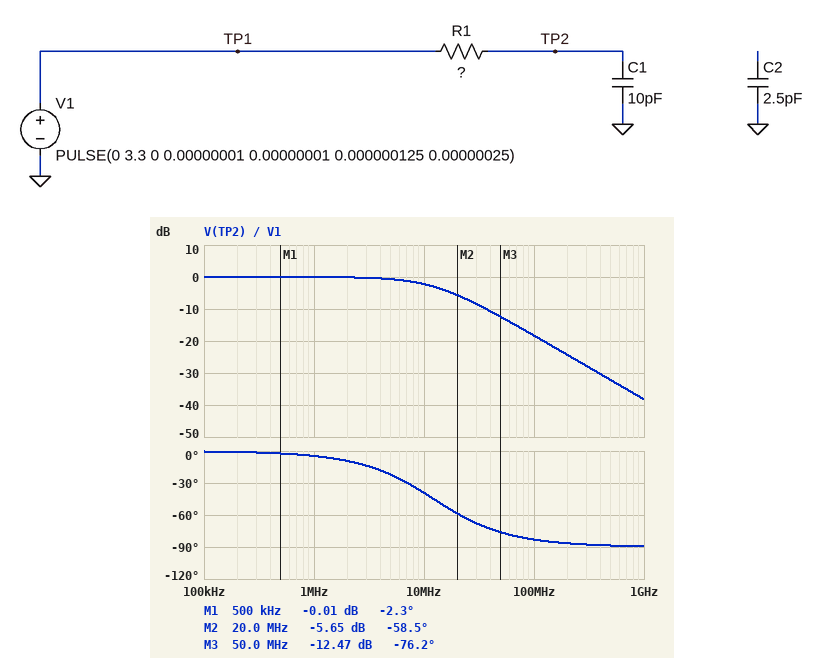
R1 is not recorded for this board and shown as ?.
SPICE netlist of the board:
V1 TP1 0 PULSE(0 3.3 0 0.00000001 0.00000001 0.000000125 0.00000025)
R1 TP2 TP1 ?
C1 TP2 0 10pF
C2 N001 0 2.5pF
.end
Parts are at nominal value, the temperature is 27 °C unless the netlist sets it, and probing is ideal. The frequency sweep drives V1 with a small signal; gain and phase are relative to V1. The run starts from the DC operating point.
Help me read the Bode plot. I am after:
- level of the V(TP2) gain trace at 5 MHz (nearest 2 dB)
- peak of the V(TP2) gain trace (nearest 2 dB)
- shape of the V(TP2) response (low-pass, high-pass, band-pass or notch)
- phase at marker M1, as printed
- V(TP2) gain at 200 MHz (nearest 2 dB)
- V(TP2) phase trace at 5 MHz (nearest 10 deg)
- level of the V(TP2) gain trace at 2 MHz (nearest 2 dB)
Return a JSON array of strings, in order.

["0 dB", "0 dB", "low-pass", "-2.3 deg", "-24 dB", "-20 deg", "0 dB"]
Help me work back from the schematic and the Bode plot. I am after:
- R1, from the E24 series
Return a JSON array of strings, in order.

["1.3 kΩ"]
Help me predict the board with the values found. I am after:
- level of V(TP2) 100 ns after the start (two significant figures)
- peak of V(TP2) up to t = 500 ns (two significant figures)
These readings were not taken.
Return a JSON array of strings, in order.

["3.3 V", "3.3 V"]
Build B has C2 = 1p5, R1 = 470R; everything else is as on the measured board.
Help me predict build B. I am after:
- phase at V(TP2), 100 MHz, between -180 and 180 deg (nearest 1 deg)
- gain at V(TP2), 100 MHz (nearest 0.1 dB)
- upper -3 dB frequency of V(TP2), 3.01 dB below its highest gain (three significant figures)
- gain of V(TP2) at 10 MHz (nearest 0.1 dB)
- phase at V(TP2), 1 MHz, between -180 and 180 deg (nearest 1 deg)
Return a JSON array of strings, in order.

["-71 deg", "-9.9 dB", "33.9 MHz", "-0.4 dB", "-2 deg"]
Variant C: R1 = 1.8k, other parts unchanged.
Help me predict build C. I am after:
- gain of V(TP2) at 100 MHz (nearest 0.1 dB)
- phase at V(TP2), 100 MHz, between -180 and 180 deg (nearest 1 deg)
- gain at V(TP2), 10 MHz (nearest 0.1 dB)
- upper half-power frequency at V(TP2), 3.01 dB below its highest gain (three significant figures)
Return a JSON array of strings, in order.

["-21.1 dB", "-85 deg", "-3.6 dB", "8.84 MHz"]
